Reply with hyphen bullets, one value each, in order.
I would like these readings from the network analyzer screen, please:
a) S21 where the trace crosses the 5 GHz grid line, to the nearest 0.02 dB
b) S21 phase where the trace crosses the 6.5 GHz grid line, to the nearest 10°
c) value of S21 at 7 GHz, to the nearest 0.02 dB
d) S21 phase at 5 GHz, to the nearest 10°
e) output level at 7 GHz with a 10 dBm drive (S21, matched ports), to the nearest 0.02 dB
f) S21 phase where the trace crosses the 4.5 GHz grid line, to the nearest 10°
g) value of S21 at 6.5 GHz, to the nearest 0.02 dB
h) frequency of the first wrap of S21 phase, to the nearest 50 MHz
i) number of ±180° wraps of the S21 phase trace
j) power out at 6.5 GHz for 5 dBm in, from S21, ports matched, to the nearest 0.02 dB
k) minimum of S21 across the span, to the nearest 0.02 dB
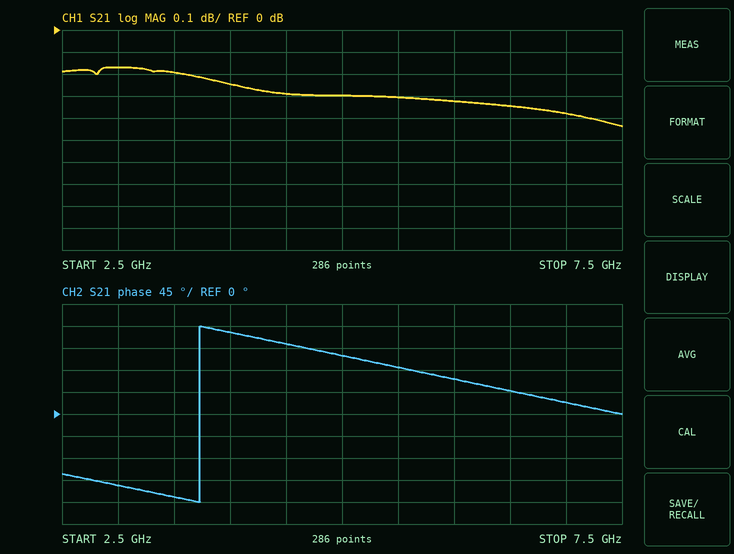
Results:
- -0.30 dB
- 50°
- -0.38 dB
- 120°
- 9.62 dBm
- 140°
- -0.34 dB
- 3.75 GHz
- 1
- 4.66 dBm
- -0.44 dB
